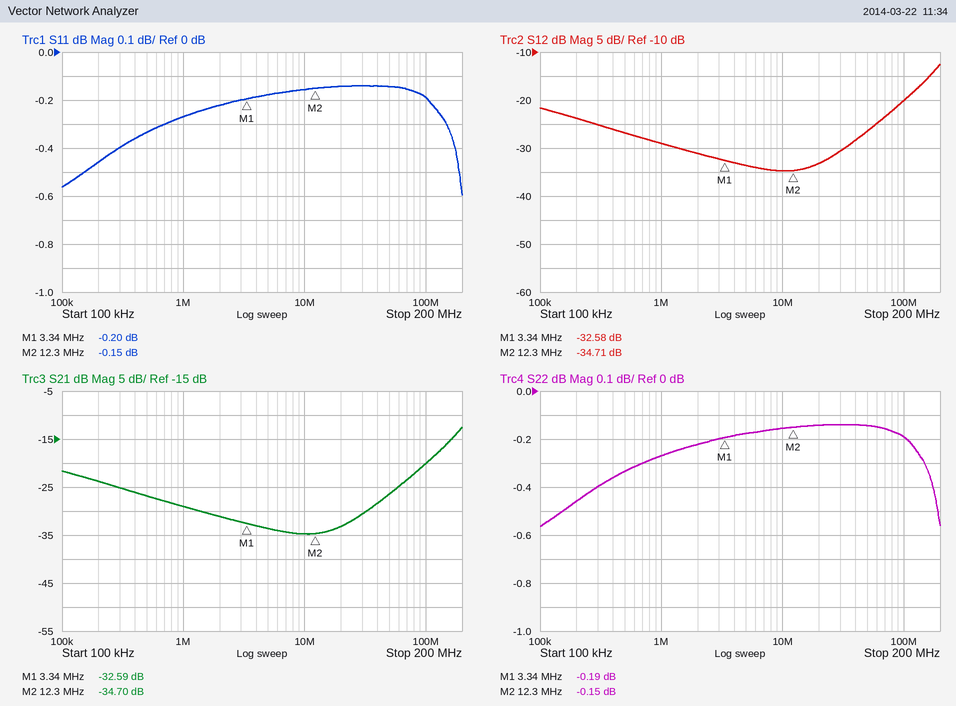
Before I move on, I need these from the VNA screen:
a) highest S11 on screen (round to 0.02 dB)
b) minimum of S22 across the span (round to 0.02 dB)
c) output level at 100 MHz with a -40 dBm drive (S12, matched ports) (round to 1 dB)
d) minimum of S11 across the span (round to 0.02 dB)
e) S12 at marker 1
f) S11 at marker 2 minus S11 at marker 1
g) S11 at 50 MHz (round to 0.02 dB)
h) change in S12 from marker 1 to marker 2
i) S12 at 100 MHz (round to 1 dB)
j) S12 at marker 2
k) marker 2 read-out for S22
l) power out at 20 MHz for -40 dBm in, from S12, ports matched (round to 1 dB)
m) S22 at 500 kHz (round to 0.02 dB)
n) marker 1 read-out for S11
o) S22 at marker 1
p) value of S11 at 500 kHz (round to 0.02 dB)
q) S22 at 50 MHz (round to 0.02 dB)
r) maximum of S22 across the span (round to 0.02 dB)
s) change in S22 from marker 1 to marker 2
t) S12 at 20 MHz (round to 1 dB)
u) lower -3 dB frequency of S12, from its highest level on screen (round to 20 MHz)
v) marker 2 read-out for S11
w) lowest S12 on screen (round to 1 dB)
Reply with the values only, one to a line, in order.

-0.14 dB
-0.56 dB
-60 dBm
-0.60 dB
-32.58 dB
0.05 dB
-0.14 dB
-2.13 dB
-20 dB
-34.71 dB
-0.15 dB
-73 dBm
-0.34 dB
-0.20 dB
-0.19 dB
-0.34 dB
-0.14 dB
-0.14 dB
0.04 dB
-33 dB
160 MHz
-0.15 dB
-35 dB
